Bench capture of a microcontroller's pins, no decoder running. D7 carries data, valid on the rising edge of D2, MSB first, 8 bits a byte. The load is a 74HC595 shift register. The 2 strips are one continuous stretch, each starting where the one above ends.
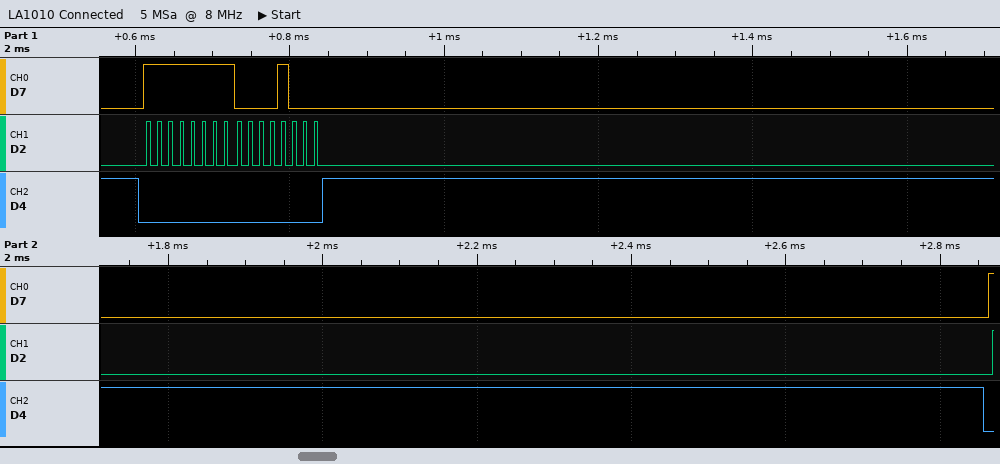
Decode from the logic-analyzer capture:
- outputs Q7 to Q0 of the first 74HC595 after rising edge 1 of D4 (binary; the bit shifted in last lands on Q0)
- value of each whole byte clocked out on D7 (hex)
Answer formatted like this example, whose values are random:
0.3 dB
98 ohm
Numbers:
00001000
FF 08
